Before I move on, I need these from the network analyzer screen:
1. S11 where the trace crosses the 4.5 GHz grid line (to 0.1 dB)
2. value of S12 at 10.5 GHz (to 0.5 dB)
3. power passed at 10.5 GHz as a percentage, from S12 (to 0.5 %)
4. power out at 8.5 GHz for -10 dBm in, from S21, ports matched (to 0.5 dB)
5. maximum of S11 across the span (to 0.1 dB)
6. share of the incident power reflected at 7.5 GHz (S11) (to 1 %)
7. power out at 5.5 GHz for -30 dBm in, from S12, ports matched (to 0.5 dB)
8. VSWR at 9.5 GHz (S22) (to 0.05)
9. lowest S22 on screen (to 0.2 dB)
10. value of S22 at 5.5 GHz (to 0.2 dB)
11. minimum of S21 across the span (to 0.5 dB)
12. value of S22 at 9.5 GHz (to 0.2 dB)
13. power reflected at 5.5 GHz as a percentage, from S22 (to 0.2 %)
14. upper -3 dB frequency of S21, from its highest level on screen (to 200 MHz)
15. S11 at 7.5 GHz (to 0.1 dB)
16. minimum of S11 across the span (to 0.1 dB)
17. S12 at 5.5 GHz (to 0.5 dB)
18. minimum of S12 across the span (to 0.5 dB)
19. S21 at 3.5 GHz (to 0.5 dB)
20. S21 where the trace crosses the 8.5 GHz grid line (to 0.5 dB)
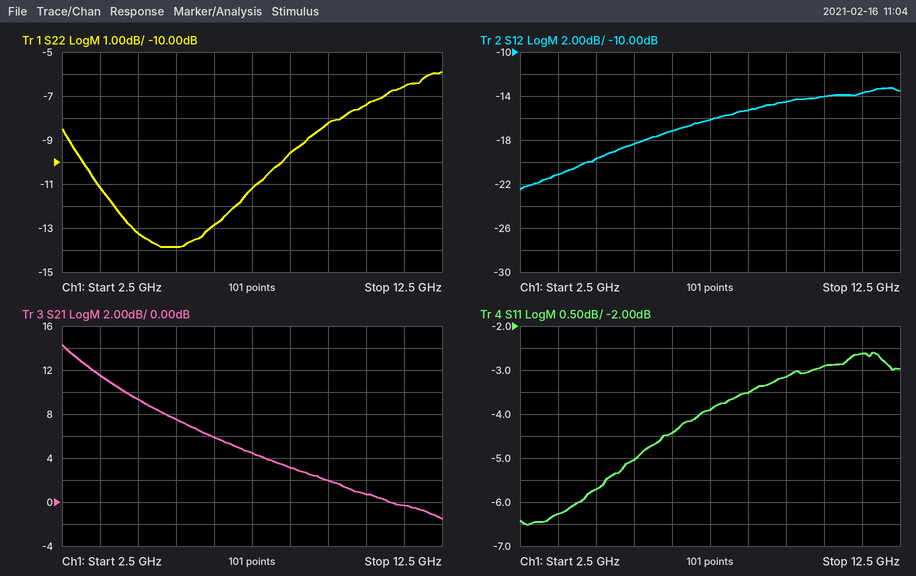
-5.7 dB
-14.0 dB
4.0 %
-7.0 dBm
-2.6 dB
41 %
-48.5 dBm
2.25
-13.8 dB
-13.8 dB
-1.5 dB
-8.2 dB
4.2 %
3.6 GHz
-3.9 dB
-6.5 dB
-18.5 dB
-22.5 dB
11.5 dB
3.0 dB
